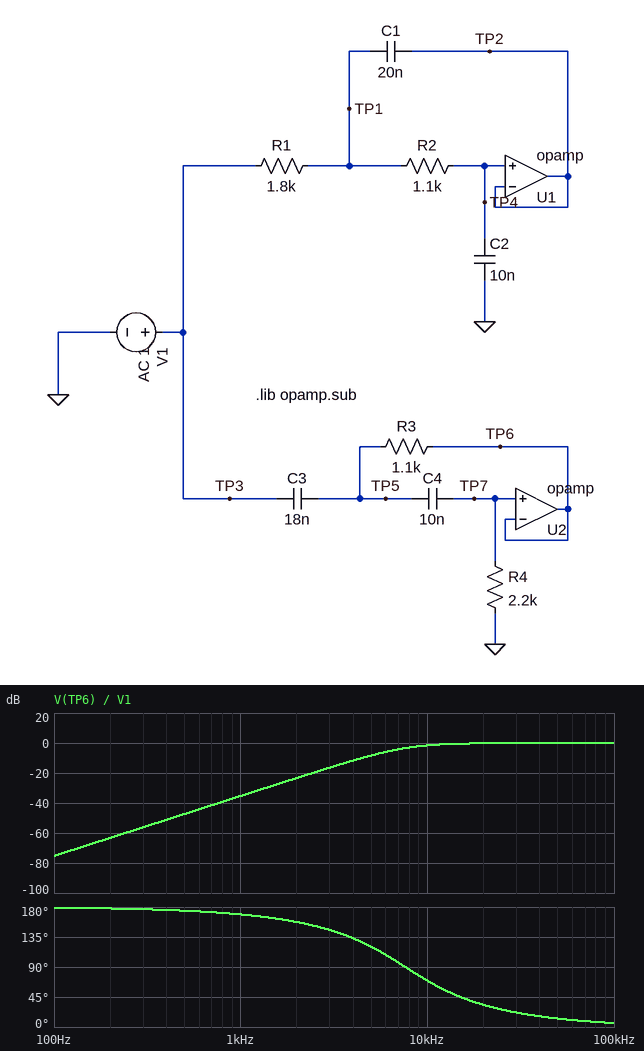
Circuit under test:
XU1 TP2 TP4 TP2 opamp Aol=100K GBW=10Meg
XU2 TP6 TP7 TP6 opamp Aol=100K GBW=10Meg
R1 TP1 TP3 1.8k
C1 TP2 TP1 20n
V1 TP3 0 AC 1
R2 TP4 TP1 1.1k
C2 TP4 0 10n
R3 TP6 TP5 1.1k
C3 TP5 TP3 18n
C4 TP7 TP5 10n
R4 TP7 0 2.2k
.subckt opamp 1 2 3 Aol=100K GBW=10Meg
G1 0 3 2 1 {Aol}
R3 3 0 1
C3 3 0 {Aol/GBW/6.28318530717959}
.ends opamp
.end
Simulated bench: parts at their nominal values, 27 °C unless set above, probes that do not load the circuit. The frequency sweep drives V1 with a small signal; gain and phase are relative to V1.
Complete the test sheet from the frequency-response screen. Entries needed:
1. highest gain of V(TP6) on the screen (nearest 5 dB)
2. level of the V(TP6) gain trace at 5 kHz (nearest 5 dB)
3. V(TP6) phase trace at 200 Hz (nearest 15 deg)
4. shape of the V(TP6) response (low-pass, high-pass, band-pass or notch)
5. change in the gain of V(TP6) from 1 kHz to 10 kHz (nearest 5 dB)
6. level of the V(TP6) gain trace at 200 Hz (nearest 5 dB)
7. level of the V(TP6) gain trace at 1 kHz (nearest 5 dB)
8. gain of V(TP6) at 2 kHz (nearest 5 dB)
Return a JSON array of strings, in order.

["0 dB", "-10 dB", "180 deg", "high-pass", "35 dB", "-65 dB", "-35 dB", "-25 dB"]
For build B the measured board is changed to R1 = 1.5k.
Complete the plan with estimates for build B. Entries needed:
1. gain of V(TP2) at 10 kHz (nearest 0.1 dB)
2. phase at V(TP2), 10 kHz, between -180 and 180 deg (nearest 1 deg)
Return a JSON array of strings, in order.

["-4.4 dB", "-101 deg"]
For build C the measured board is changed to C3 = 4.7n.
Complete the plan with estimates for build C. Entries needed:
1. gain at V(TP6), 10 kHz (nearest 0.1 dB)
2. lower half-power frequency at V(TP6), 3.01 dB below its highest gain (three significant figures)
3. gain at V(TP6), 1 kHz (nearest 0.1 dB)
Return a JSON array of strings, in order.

["-8.2 dB", "16.0 kHz", "-47.0 dB"]
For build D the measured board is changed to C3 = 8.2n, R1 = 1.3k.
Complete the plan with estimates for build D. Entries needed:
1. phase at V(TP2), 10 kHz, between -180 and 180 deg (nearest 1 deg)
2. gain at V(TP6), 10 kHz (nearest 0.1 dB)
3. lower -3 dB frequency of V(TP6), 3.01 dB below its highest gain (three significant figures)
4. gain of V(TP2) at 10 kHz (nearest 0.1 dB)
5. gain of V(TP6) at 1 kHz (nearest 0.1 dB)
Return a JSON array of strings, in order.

["-95 deg", "-4.2 dB", "11.3 kHz", "-3.6 dB", "-42.1 dB"]
